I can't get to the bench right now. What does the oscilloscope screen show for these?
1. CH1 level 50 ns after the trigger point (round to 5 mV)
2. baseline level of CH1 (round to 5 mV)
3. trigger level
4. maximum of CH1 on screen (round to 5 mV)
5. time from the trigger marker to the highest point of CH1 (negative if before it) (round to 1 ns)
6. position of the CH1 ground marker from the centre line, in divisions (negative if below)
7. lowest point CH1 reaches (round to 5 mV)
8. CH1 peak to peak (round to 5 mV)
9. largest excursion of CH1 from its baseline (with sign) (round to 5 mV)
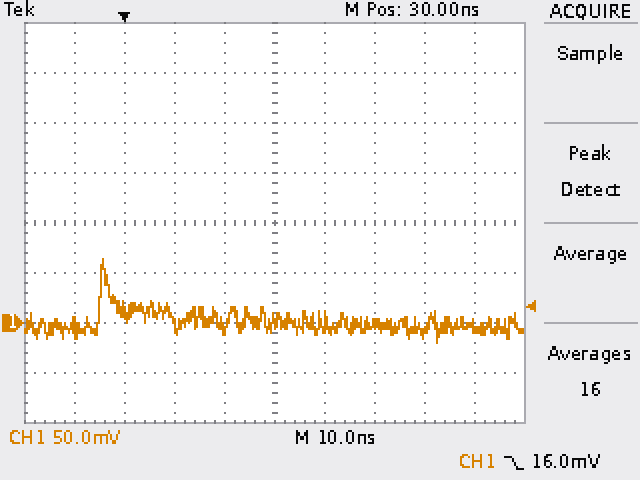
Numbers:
0 mV
0 mV
16.0 mV
65 mV
-4 ns
-2.0 div
-20 mV
85 mV
+65 mV
